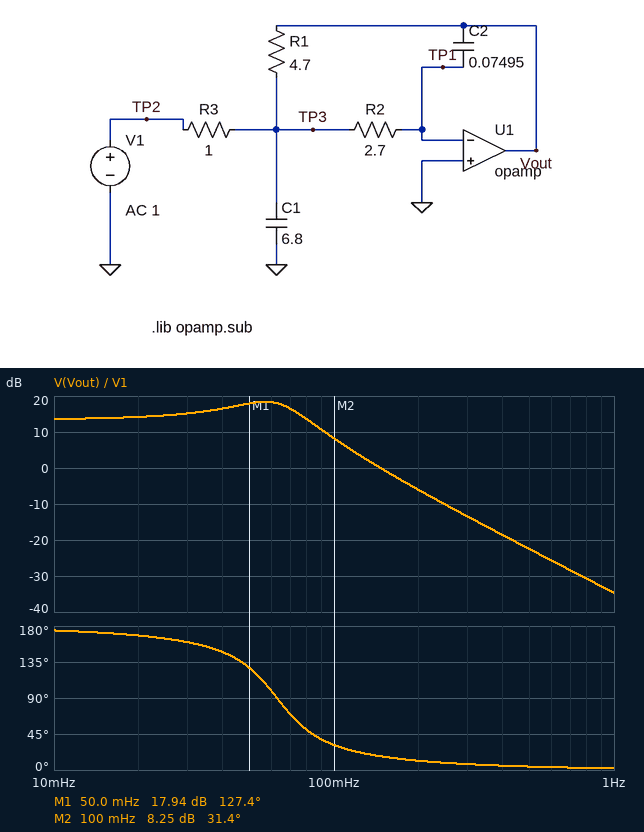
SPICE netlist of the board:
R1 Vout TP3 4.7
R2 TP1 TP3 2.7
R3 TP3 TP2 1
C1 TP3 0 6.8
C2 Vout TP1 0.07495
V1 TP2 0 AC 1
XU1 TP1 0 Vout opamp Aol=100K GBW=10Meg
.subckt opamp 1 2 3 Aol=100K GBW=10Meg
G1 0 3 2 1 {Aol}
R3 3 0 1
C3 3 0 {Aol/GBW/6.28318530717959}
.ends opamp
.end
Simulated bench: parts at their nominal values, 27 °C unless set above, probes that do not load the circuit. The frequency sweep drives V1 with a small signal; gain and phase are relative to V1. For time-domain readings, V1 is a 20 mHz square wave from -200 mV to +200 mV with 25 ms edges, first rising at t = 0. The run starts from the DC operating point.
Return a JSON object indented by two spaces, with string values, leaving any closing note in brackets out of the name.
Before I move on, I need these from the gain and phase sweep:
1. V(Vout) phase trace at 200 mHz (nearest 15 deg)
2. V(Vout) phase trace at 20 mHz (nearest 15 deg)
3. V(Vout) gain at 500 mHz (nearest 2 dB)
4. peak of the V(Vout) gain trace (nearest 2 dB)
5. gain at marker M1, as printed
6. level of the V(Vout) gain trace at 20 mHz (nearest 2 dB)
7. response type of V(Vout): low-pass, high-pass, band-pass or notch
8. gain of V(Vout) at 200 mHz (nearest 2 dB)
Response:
{
  "V(Vout) phase trace at 200 mHz": "15 deg",
  "V(Vout) phase trace at 20 mHz": "165 deg",
  "V(Vout) gain at 500 mHz": "-22 dB",
  "peak of the V(Vout) gain trace": "18 dB",
  "gain at marker M1, as printed": "17.94 dB",
  "level of the V(Vout) gain trace at 20 mHz": "14 dB",
  "response type of V(Vout): low-pass, high-pass, band-pass or notch": "low-pass",
  "gain of V(Vout) at 200 mHz": "-6 dB"
}
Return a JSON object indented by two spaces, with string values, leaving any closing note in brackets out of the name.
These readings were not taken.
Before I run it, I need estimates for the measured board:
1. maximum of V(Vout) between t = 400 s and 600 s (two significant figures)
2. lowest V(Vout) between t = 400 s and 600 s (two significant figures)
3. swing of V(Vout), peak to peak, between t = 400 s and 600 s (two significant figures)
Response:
{
  "maximum of V(Vout) between t = 400 s and 600 s": "1.7 V",
  "lowest V(Vout) between t = 400 s and 600 s": "-1.7 V",
  "swing of V(Vout), peak to peak, between t = 400 s and 600 s": "3.4 V"
}
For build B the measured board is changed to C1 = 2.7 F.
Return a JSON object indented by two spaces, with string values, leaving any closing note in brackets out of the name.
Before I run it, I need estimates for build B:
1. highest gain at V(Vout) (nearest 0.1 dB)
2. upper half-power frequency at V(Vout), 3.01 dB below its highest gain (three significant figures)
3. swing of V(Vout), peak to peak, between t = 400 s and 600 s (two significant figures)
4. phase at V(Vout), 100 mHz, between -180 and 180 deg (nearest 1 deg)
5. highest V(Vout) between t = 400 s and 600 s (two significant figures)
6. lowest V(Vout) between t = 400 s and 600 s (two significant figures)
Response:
{
  "highest gain at V(Vout)": "15.1 dB",
  "upper half-power frequency at V(Vout), 3.01 dB below its highest gain": "117 mHz",
  "swing of V(Vout), peak to peak, between t = 400 s and 600 s": "2.6 V",
  "phase at V(Vout), 100 mHz, between -180 and 180 deg": "89 deg",
  "highest V(Vout) between t = 400 s and 600 s": "1.3 V",
  "lowest V(Vout) between t = 400 s and 600 s": "-1.3 V"
}
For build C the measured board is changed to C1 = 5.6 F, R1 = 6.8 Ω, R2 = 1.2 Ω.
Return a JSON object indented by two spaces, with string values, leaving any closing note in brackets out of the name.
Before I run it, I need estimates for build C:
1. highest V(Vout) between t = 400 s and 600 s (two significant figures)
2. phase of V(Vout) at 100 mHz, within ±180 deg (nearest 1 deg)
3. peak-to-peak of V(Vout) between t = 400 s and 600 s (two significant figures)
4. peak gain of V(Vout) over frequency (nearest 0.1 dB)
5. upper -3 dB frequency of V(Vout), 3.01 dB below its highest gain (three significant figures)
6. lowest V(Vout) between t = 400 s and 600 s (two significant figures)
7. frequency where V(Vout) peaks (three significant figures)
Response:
{
  "highest V(Vout) between t = 400 s and 600 s": "2.3 V",
  "phase of V(Vout) at 100 mHz, within ±180 deg": "65 deg",
  "peak-to-peak of V(Vout) between t = 400 s and 600 s": "4.5 V",
  "peak gain of V(Vout) over frequency": "20.8 dB",
  "upper -3 dB frequency of V(Vout), 3.01 dB below its highest gain": "102 mHz",
  "lowest V(Vout) between t = 400 s and 600 s": "-2.3 V",
  "frequency where V(Vout) peaks": "76.2 mHz"
}
